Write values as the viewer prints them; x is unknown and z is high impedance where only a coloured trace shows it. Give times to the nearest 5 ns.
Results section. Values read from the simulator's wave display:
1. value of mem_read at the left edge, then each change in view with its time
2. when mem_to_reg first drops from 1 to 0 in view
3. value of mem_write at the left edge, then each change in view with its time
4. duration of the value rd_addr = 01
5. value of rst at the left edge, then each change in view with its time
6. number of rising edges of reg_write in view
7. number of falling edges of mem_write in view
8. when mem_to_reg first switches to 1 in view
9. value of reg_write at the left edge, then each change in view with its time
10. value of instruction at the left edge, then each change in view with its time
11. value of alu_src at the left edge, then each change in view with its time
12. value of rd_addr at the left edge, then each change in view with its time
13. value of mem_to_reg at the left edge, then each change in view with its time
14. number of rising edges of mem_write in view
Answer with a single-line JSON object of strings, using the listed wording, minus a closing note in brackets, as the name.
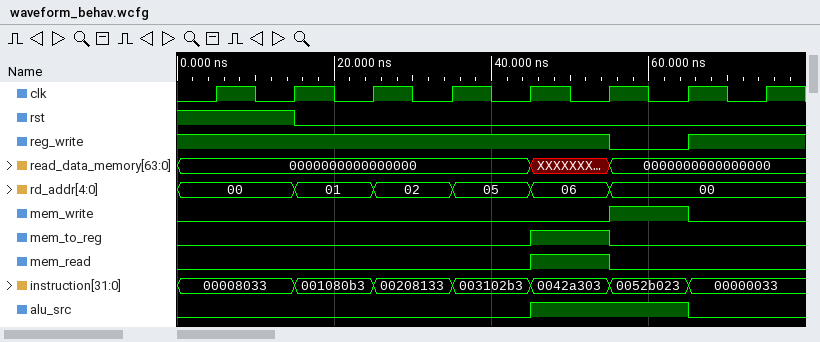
{"value of mem_read at the left edge, then each change in view with its time": "0, 1 at 45 ns, 0 at 55 ns", "when mem_to_reg first drops from 1 to 0 in view": "55 ns", "value of mem_write at the left edge, then each change in view with its time": "0, 1 at 55 ns, 0 at 65 ns", "duration of the value rd_addr = 01": "10 ns", "value of rst at the left edge, then each change in view with its time": "1, 0 at 15 ns", "number of rising edges of reg_write in view": "1", "number of falling edges of mem_write in view": "1", "when mem_to_reg first switches to 1 in view": "45 ns", "value of reg_write at the left edge, then each change in view with its time": "1, 0 at 55 ns, 1 at 65 ns", "value of instruction at the left edge, then each change in view with its time": "00008033, 001080b3 at 15 ns, 00208133 at 25 ns, 003102b3 at 35 ns, 0042a303 at 45 ns, 0052b023 at 55 ns, 00000033 at 65 ns", "value of alu_src at the left edge, then each change in view with its time": "0, 1 at 45 ns, 0 at 65 ns", "value of rd_addr at the left edge, then each change in view with its time": "00, 01 at 15 ns, 02 at 25 ns, 05 at 35 ns, 06 at 45 ns, 00 at 55 ns", "value of mem_to_reg at the left edge, then each change in view with its time": "0, 1 at 45 ns, 0 at 55 ns", "number of rising edges of mem_write in view": "1"}
